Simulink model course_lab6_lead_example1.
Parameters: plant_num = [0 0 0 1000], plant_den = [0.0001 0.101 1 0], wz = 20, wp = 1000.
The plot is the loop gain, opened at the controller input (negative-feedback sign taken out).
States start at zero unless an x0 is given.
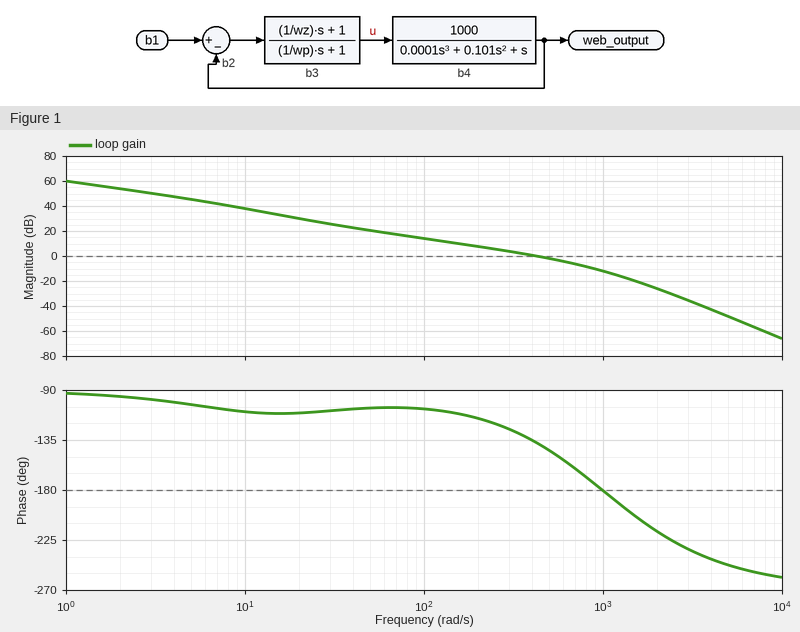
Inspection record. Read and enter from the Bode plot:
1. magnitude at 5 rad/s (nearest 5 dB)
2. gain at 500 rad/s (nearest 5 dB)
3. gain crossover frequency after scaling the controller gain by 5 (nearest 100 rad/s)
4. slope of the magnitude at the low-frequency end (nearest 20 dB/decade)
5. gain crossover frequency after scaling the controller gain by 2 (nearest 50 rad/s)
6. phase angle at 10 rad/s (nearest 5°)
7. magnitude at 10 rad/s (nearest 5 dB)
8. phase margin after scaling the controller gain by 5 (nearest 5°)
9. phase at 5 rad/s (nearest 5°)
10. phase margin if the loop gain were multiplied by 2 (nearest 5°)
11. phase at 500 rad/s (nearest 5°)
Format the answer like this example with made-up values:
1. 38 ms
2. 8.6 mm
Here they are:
1. 45 dB
2. 0 dB
3. 1100 rad/s
4. -20 dB/decade
5. 700 rad/s
6. -110°
7. 40 dB
8. -5°
9. -105°
10. 20°
11. -145°
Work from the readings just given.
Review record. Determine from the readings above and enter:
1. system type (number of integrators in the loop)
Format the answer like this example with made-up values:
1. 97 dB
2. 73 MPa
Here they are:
1. 1
